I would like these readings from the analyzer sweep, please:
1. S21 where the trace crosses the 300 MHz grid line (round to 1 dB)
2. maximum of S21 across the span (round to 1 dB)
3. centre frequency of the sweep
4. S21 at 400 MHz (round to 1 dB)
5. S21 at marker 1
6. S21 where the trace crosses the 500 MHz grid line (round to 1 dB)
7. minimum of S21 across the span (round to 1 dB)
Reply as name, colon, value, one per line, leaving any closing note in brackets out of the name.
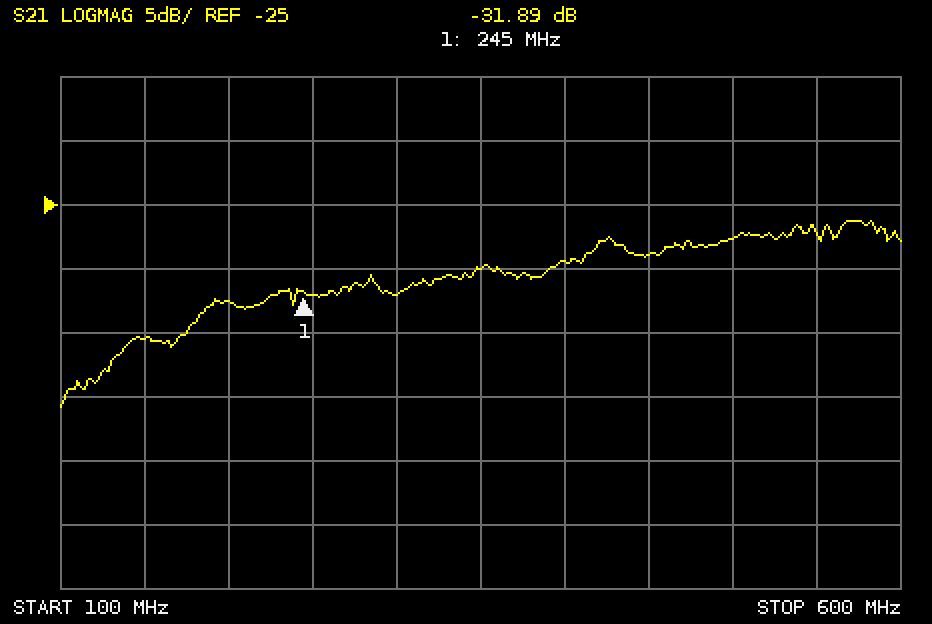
S21 where the trace crosses the 300 MHz grid line: -32 dB
maximum of S21 across the span: -26 dB
centre frequency of the sweep: 350 MHz
S21 at 400 MHz: -29 dB
S21 at marker 1: -31.89 dB
S21 where the trace crosses the 500 MHz grid line: -28 dB
minimum of S21 across the span: -41 dB
